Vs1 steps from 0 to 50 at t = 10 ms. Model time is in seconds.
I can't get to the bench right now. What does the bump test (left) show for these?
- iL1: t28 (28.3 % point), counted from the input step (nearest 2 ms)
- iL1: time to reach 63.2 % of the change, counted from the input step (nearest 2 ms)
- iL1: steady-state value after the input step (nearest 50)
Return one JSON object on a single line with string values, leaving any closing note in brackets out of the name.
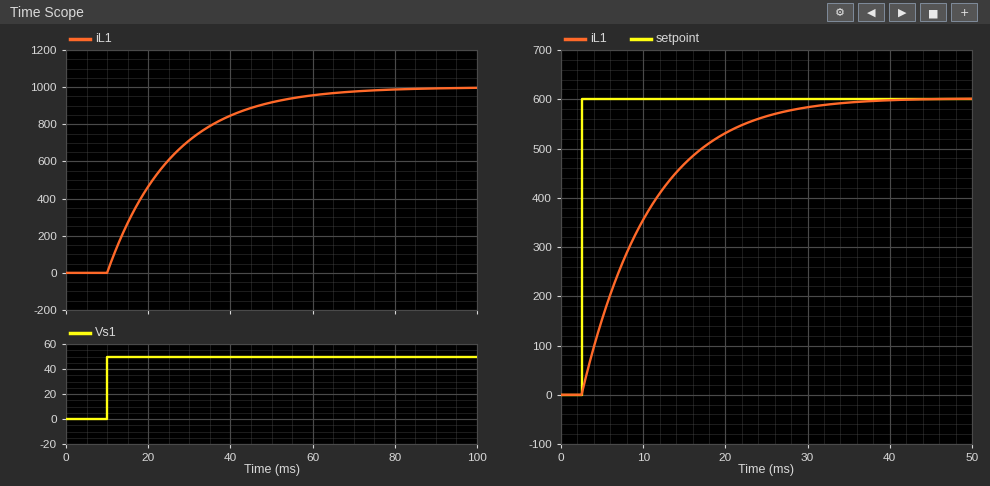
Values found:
{"iL1: t28 (28.3 % point), counted from the input step": "6 ms", "iL1: time to reach 63.2 % of the change, counted from the input step": "16 ms", "iL1: steady-state value after the input step": "1000"}
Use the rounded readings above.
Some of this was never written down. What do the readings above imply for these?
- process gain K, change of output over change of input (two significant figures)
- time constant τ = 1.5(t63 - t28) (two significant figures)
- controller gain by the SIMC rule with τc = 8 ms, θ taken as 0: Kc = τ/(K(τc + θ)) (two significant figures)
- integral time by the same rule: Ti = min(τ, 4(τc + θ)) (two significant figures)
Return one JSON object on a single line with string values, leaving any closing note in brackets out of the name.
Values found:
{"process gain K, change of output over change of input": "20", "time constant τ = 1.5(t63 - t28)": "15 ms", "controller gain by the SIMC rule with τc = 8 ms, θ taken as 0: Kc = τ/(K(τc + θ))": "0.094", "integral time by the same rule: Ti = min(τ, 4(τc + θ))": "15 ms"}
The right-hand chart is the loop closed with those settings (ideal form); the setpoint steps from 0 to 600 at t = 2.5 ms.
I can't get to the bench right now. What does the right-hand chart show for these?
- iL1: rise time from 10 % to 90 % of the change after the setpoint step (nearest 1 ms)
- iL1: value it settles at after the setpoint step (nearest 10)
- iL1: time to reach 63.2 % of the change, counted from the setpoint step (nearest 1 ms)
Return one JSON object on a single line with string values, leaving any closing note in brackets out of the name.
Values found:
{"iL1: rise time from 10 % to 90 % of the change after the setpoint step": "18 ms", "iL1: value it settles at after the setpoint step": "600", "iL1: time to reach 63.2 % of the change, counted from the setpoint step": "8 ms"}
